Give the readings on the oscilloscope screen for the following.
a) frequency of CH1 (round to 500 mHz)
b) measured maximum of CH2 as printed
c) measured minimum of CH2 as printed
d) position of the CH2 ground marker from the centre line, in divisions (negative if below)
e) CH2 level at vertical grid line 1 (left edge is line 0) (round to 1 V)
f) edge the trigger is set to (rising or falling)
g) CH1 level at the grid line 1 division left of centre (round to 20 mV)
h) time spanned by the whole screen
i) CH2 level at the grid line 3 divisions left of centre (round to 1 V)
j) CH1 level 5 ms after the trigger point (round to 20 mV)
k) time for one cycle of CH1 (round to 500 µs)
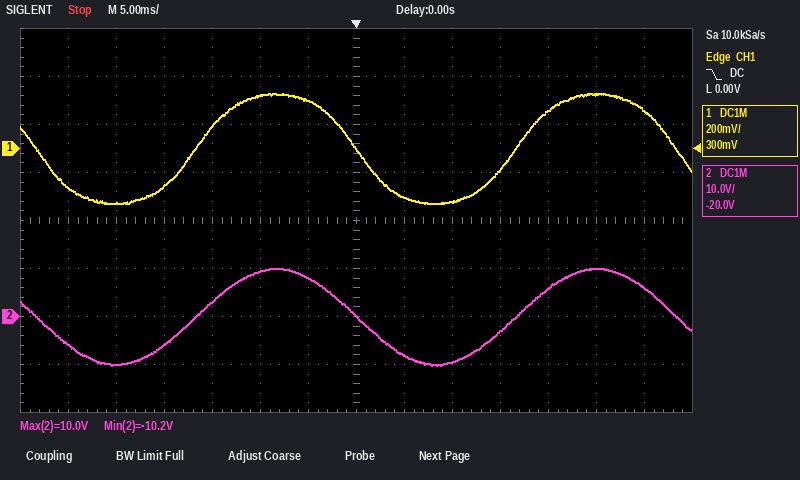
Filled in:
30.0 Hz
10.0 V
-10.2 V
-2.0 div
-6 V
falling
200 mV
70 ms
3 V
-200 mV
33.5 ms
